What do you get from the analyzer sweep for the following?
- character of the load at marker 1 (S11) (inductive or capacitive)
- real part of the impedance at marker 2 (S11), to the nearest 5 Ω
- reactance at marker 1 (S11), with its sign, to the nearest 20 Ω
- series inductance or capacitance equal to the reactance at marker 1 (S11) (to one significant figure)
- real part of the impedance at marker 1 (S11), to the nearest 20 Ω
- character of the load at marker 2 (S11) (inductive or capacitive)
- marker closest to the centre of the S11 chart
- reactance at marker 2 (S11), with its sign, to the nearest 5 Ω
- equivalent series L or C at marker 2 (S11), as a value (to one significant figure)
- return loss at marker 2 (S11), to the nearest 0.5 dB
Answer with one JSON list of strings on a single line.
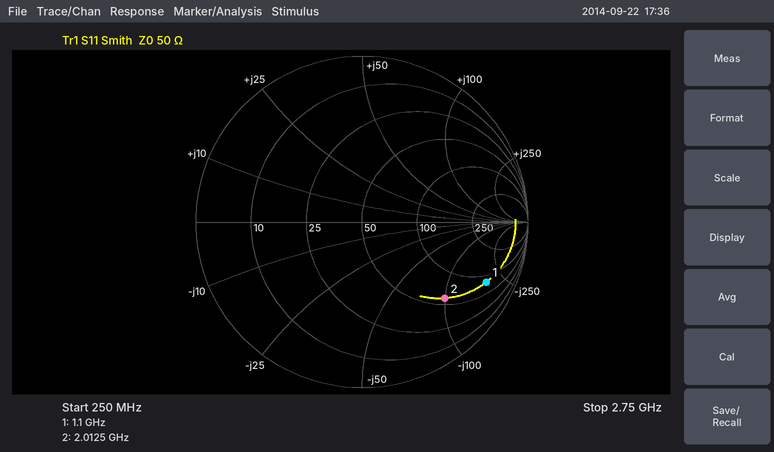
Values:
["capacitive", "60 Ω", "-180 Ω", "800 fF", "80 Ω", "capacitive", "marker 2", "-100 Ω", "800 fF", "3.5 dB"]
